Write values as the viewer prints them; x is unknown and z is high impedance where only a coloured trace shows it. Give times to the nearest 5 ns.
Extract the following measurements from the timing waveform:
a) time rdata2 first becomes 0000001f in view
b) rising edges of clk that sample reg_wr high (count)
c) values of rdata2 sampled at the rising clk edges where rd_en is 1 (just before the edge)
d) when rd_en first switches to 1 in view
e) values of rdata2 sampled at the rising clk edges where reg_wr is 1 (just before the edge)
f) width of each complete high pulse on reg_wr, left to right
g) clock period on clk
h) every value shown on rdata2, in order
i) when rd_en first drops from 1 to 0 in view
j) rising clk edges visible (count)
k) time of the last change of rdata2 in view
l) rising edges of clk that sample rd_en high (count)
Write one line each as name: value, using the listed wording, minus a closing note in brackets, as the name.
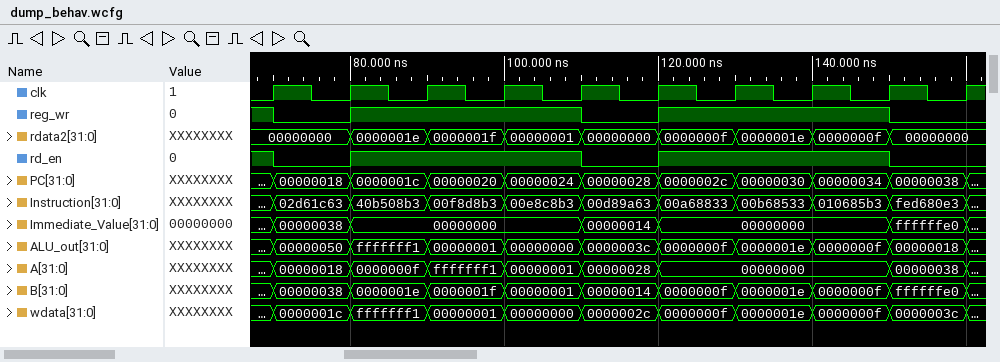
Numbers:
time rdata2 first becomes 0000001f in view: 90 ns
rising edges of clk that sample reg_wr high: 7
values of rdata2 sampled at the rising clk edges where rd_en is 1: 00000000, 0000001e, 0000001f, 00000001, 0000000f, 0000001e, 0000000f
when rd_en first switches to 1 in view: 80 ns
values of rdata2 sampled at the rising clk edges where reg_wr is 1: 00000000, 0000001e, 0000001f, 00000001, 0000000f, 0000001e, 0000000f
width of each complete high pulse on reg_wr, left to right: 30 ns, 30 ns
clock period on clk: 10 ns
every value shown on rdata2, in order: 00000000, 0000001e, 0000001f, 00000001, 00000000, 0000000f, 0000001e, 0000000f, 00000000
when rd_en first drops from 1 to 0 in view: 70 ns
rising clk edges visible: 10
time of the last change of rdata2 in view: 150 ns
rising edges of clk that sample rd_en high: 7
